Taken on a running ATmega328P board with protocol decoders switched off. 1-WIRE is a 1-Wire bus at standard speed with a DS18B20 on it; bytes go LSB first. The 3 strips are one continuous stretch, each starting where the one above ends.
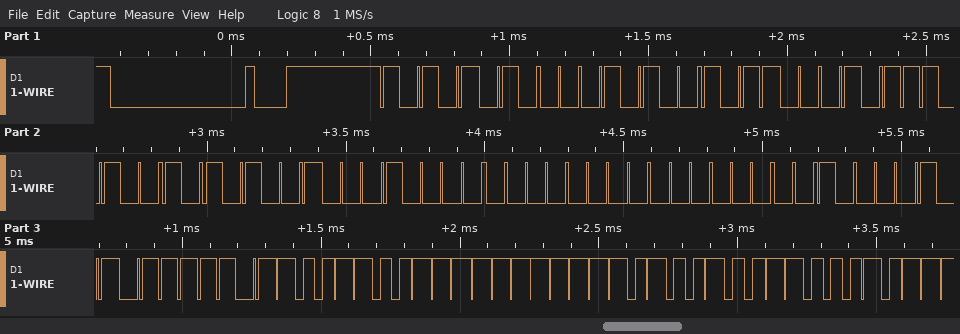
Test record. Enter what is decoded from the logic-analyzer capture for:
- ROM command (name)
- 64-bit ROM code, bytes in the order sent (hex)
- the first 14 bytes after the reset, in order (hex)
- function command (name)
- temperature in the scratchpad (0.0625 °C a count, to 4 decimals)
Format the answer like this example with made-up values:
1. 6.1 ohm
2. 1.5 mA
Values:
1. Match ROM
2. 28 8D 2E 95 08 00 00 A1
3. 55 28 8D 2E 95 08 00 00 A1 BE 99 FF 4B 46
4. Read Scratchpad
5. -6.4375 °C
